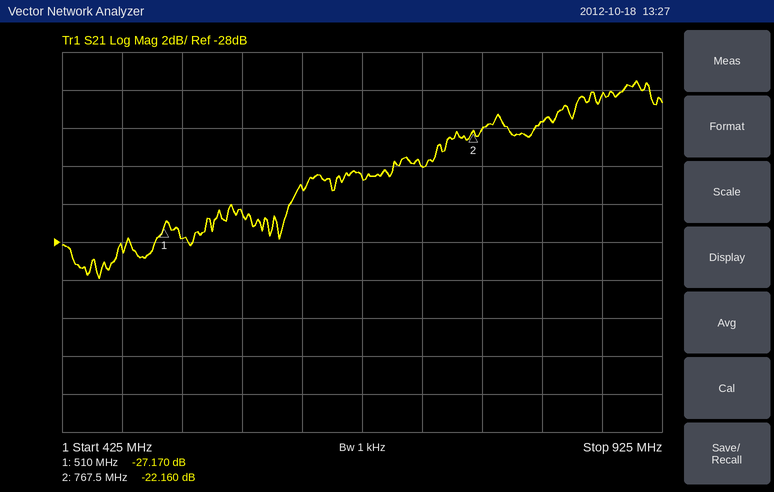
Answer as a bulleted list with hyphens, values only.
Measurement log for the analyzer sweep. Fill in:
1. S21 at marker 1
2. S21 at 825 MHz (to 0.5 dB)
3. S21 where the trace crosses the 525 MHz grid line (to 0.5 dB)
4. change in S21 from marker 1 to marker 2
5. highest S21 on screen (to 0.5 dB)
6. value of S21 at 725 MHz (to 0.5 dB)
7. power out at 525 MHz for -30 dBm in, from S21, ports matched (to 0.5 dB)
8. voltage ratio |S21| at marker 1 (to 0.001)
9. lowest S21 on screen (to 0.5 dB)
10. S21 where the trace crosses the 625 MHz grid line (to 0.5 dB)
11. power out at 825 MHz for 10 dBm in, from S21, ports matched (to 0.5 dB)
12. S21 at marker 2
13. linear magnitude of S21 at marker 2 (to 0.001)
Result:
- -27.170 dB
- -21.5 dB
- -28.0 dB
- 5.010 dB
- -19.5 dB
- -24.0 dB
- -58.0 dBm
- 0.044
- -30.0 dB
- -25.0 dB
- -11.5 dBm
- -22.160 dB
- 0.078
